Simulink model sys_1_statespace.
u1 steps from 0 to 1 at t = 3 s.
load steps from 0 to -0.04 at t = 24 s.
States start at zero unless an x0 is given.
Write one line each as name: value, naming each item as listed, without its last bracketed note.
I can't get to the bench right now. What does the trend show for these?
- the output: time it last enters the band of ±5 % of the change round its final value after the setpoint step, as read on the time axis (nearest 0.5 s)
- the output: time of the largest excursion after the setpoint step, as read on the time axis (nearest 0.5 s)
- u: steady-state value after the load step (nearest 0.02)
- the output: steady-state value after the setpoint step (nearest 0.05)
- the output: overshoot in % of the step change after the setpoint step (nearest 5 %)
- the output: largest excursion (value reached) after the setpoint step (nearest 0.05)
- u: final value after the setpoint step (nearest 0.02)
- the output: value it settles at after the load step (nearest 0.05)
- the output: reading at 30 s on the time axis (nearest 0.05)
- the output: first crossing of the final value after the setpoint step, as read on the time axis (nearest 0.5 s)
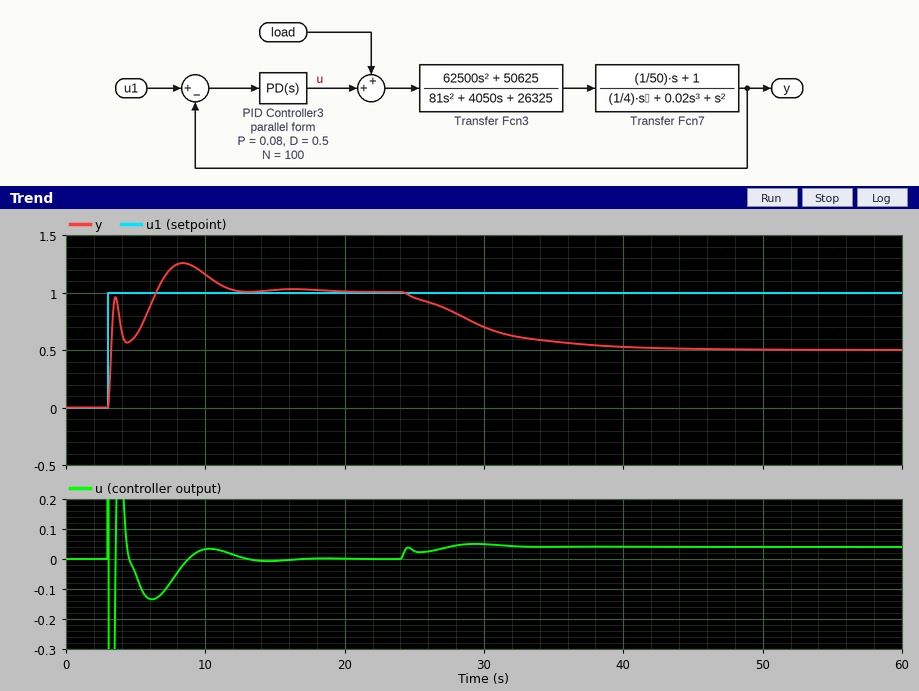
the output: time it last enters the band of ±5 % of the change round its final value after the setpoint step, as read on the time axis: 11.5 s
the output: time of the largest excursion after the setpoint step, as read on the time axis: 8.5 s
u: steady-state value after the load step: 0.04
the output: steady-state value after the setpoint step: 1.00
the output: overshoot in % of the step change after the setpoint step: 25 %
the output: largest excursion (value reached) after the setpoint step: 1.25
u: final value after the setpoint step: 0.00
the output: value it settles at after the load step: 0.50
the output: reading at 30 s on the time axis: 0.70
the output: first crossing of the final value after the setpoint step, as read on the time axis: 6.5 s
